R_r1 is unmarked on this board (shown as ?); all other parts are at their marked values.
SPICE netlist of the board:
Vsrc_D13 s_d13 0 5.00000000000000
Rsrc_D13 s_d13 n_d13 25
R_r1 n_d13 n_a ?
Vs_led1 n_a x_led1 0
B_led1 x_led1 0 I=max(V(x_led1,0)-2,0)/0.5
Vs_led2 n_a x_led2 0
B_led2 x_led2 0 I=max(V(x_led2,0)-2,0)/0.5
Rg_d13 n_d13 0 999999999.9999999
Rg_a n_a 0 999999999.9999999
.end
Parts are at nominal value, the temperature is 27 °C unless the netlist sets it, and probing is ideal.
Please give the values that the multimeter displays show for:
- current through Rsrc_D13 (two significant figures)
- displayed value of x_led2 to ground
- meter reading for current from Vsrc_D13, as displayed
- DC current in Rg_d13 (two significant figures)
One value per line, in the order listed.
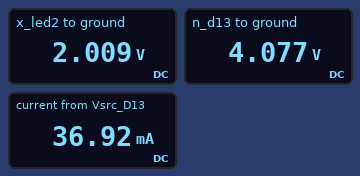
37 mA
2.009 V
36.92 mA
4.1 nA
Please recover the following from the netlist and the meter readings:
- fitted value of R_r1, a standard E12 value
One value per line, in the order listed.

56 Ω
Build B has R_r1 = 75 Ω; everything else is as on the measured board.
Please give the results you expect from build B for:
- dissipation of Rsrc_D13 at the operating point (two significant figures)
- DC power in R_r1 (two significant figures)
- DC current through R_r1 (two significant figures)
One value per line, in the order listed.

22 mW
67 mW
30 mA
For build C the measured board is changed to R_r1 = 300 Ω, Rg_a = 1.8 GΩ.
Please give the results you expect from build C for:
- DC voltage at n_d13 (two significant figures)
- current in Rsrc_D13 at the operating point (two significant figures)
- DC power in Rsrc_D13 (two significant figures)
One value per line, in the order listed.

4.8 V
9.2 mA
2.1 mW
